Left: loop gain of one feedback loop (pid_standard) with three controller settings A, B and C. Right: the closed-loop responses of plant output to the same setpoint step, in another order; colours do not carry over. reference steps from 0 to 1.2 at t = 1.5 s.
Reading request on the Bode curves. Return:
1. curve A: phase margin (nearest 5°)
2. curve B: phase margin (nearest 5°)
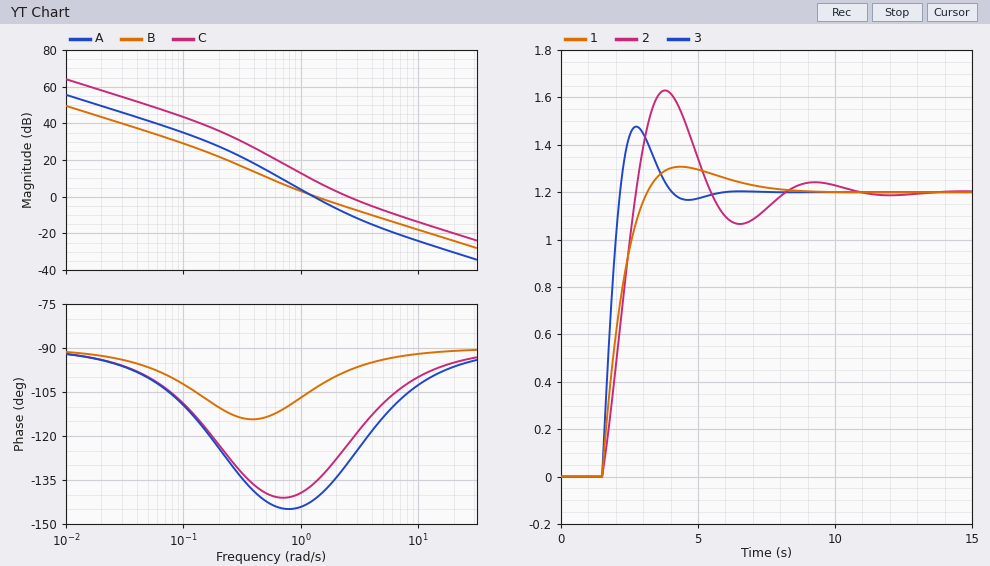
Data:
40°
75°
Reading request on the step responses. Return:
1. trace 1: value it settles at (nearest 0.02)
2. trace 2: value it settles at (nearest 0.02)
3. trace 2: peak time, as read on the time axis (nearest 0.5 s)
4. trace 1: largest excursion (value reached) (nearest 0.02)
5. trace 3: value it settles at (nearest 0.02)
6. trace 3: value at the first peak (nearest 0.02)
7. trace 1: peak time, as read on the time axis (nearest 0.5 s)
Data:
1.20
1.20
4.0 s
1.30
1.20
1.48
4.5 s
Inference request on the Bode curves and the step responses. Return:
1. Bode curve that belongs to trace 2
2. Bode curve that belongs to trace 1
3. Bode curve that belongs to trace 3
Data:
A
B
C
